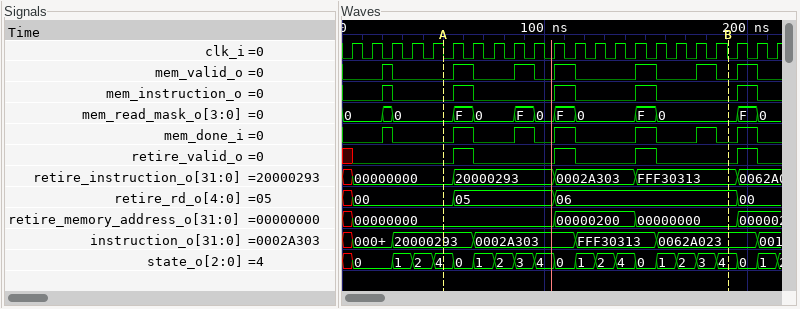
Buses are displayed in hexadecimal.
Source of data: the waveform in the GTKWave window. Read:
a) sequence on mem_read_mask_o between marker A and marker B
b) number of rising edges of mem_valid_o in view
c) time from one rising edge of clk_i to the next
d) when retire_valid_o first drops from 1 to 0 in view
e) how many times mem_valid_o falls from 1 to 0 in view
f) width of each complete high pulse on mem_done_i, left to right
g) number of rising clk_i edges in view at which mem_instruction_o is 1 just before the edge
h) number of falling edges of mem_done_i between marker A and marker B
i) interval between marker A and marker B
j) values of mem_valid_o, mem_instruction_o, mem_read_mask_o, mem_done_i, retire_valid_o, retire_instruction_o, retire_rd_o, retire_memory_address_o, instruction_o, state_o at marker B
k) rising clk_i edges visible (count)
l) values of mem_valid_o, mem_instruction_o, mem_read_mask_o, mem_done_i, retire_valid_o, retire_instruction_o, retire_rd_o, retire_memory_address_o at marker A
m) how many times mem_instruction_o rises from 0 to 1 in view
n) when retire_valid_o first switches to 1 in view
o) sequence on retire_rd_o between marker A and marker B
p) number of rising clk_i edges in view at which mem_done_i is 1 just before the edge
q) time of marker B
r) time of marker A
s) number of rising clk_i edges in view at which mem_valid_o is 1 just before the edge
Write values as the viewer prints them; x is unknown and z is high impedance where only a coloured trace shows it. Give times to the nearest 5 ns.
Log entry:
0, F, 0, F, 0, F, 0, F, 0
7
10 ns
65 ns
7
5 ns, 10 ns, 10 ns, 10 ns, 10 ns, 10 ns, 10 ns
5
5
140 ns
mem_valid_o=0, mem_instruction_o=0, mem_read_mask_o=0, mem_done_i=0, retire_valid_o=0, retire_instruction_o=FFF30313, retire_rd_o=06, retire_memory_address_o=00000000, instruction_o=0062A023, state_o=4
22
mem_valid_o=0, mem_instruction_o=0, mem_read_mask_o=0, mem_done_i=0, retire_valid_o=0, retire_instruction_o=00000000, retire_rd_o=00, retire_memory_address_o=00000000
5
55 ns
00, 05, 06
7
190 ns
50 ns
7
